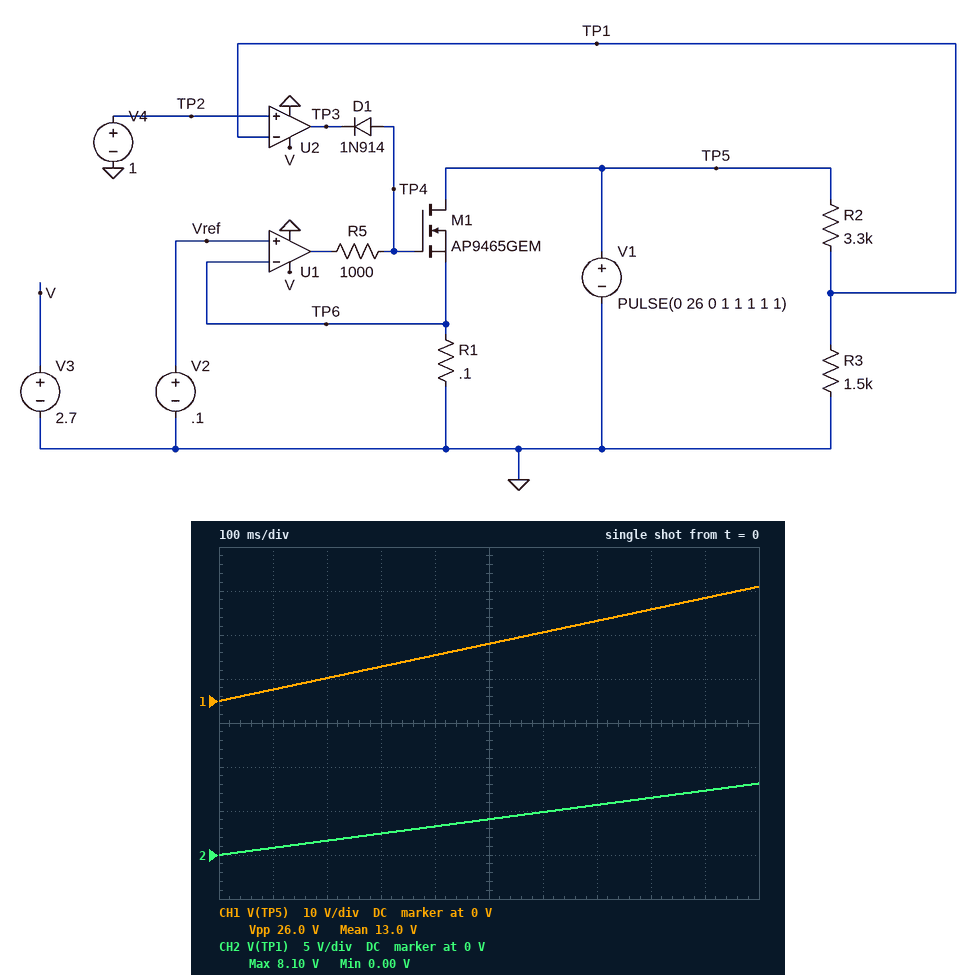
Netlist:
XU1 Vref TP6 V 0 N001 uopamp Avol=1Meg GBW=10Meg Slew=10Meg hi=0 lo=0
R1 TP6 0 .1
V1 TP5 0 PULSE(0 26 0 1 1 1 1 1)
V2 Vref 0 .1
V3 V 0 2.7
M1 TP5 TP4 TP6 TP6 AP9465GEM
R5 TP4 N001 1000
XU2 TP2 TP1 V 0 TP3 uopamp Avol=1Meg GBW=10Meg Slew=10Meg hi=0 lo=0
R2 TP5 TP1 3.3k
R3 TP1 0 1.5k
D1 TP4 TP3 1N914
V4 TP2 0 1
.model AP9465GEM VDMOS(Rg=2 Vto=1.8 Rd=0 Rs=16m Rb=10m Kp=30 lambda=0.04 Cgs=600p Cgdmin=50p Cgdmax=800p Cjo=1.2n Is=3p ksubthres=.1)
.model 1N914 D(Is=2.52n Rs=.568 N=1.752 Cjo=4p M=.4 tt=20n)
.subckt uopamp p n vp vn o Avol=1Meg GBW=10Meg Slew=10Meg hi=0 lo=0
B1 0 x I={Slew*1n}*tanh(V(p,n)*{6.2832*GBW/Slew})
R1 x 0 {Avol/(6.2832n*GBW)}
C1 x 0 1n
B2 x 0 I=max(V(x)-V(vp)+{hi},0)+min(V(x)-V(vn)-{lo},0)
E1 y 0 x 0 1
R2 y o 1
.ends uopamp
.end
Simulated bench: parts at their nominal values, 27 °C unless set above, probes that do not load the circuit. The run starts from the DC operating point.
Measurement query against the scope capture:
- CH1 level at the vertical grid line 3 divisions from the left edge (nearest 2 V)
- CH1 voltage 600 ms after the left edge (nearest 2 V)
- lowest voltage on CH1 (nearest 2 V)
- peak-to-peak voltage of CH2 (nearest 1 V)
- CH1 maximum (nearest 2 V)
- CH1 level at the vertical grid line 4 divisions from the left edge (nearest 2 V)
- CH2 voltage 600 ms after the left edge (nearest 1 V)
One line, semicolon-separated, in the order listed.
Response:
8 V; 16 V; 0 V; 8 V; 26 V; 10 V; 5 V
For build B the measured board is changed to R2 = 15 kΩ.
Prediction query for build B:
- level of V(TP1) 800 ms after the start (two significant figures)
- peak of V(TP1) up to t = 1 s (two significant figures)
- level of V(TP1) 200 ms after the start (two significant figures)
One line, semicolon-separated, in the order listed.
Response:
1.9 V; 2.4 V; 470 mV
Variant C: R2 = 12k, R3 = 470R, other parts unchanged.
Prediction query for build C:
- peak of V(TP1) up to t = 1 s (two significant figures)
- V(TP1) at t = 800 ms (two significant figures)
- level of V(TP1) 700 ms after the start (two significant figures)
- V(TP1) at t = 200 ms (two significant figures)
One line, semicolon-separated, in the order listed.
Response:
980 mV; 780 mV; 690 mV; 200 mV
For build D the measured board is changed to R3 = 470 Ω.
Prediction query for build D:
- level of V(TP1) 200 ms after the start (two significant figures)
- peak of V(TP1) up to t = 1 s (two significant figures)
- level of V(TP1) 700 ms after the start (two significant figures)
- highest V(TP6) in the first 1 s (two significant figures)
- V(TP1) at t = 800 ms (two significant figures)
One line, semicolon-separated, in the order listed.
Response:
650 mV; 3.2 V; 2.3 V; 100 mV; 2.6 V
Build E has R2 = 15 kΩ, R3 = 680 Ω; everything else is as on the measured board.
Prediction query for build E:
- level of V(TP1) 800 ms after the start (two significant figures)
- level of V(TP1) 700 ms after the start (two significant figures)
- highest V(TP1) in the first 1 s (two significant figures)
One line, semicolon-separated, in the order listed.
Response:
900 mV; 790 mV; 1.1 V
